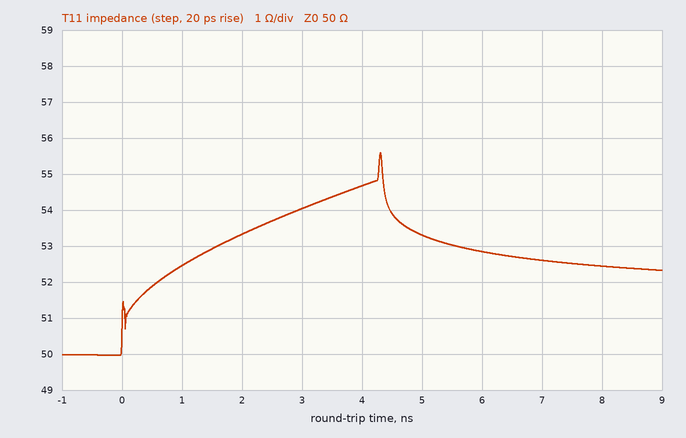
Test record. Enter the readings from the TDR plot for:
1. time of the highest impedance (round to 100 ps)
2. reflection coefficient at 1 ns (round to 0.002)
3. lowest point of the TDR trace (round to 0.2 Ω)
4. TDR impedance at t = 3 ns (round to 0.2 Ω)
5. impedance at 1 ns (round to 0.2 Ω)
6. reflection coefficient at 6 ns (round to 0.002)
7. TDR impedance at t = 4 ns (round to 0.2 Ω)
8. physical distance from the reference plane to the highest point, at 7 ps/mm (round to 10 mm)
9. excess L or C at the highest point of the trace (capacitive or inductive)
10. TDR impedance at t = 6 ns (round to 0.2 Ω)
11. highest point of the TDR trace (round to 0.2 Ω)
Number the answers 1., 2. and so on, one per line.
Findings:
1. 4.3 ns
2. +0.024
3. 50.0 Ω
4. 54.0 Ω
5. 52.4 Ω
6. +0.028
7. 54.6 Ω
8. 310 mm
9. inductive
10. 52.8 Ω
11. 55.6 Ω
